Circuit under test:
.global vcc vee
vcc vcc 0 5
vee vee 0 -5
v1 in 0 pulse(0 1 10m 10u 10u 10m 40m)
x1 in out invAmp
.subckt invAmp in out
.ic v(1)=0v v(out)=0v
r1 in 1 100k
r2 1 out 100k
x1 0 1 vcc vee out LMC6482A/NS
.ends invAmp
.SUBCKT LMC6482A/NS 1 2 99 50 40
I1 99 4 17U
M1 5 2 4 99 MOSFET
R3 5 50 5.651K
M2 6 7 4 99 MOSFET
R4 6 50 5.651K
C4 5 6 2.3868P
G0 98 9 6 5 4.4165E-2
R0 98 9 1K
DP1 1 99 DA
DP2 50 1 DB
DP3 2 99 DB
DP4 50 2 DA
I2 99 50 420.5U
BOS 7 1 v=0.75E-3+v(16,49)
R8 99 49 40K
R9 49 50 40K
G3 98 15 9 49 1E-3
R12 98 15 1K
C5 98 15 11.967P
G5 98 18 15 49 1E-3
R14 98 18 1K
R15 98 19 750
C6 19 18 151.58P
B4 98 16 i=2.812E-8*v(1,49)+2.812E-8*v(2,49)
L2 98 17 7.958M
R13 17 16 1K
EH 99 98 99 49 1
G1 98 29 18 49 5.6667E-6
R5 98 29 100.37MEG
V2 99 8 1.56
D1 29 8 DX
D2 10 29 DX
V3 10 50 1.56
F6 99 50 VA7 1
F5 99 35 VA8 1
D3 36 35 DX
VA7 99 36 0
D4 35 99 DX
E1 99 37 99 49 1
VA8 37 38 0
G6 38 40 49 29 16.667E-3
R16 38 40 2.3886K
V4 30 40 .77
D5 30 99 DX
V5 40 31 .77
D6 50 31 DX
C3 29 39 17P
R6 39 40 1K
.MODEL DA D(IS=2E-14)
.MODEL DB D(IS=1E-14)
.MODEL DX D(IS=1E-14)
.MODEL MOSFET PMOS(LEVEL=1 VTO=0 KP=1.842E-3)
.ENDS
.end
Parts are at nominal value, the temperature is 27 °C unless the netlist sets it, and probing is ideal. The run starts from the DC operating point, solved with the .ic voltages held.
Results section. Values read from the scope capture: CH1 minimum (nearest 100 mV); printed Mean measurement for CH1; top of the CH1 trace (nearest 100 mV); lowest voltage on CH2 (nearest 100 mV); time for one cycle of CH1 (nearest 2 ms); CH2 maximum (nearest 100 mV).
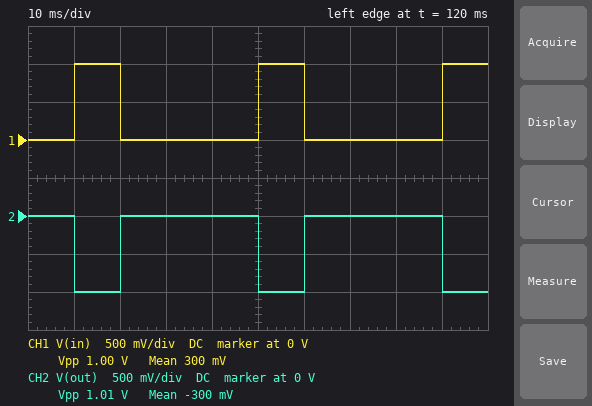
0 V
300 mV
1.0 V
-1.0 V
40 ms
0 V
